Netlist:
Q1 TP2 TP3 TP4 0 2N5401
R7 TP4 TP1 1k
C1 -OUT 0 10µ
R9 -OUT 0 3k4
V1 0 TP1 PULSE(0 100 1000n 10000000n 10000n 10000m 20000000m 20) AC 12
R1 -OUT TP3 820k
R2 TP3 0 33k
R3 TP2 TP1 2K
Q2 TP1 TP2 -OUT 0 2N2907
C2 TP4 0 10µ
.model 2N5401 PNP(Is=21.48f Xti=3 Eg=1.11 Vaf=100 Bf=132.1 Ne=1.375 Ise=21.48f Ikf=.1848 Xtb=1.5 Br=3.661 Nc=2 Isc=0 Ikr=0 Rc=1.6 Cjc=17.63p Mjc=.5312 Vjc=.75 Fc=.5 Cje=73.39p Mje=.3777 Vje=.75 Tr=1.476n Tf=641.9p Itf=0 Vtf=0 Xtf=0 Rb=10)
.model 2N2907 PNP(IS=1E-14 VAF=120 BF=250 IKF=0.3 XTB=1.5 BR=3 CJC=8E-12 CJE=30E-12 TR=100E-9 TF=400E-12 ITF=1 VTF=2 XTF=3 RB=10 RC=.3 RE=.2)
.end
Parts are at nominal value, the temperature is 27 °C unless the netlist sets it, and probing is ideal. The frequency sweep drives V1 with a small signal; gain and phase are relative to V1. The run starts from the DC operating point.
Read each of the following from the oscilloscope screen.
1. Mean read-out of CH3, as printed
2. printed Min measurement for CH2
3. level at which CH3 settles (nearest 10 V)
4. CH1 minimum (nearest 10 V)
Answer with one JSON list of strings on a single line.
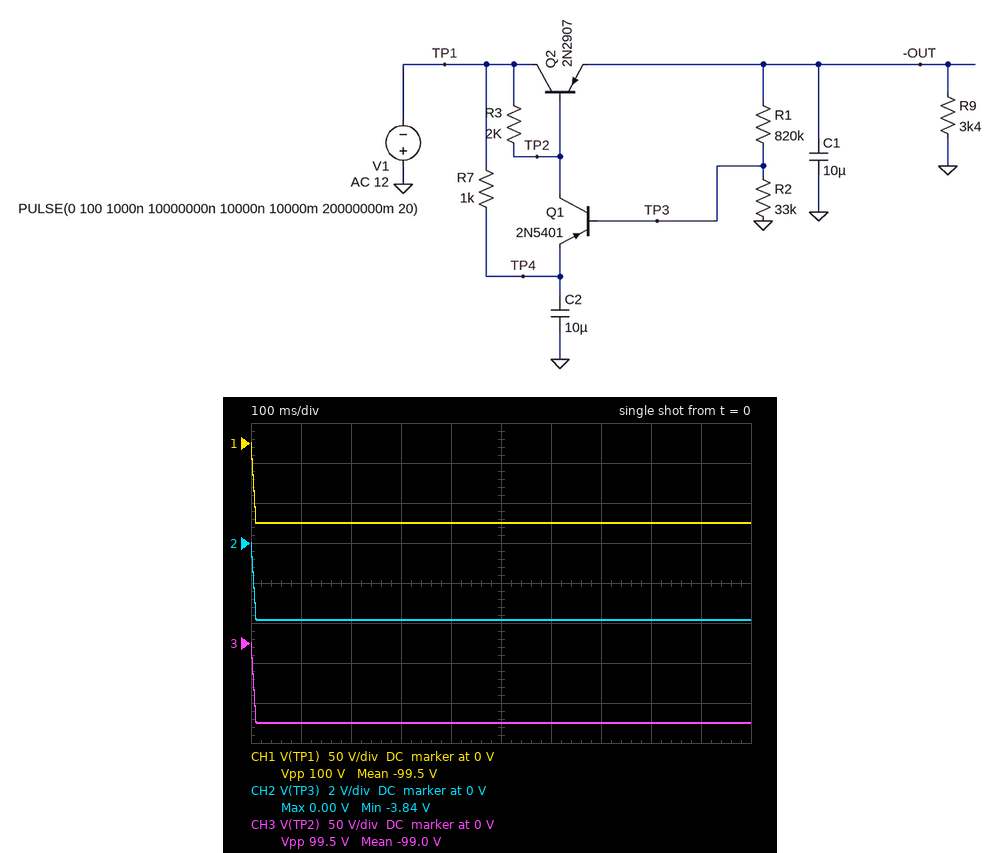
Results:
["-99.0 V", "-3.84 V", "-100 V", "-100 V"]
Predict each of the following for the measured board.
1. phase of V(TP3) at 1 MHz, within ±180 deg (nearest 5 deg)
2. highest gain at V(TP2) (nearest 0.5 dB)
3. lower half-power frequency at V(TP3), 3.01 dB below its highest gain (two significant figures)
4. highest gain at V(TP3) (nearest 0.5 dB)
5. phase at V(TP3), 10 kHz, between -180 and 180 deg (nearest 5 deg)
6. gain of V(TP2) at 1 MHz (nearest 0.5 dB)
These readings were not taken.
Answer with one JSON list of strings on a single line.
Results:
["155 deg", "0 dB", "51 kHz", "-14.5 dB", "-100 deg", "-1.5 dB"]
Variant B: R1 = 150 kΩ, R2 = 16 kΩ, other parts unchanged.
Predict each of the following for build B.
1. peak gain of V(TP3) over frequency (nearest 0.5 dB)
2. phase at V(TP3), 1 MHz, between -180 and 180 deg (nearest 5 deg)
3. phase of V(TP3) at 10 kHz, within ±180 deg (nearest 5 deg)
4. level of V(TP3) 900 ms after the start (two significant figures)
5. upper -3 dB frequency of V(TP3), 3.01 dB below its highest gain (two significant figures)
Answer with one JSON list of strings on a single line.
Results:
["-15.0 dB", "160 deg", "-95 deg", "-9.5 V", "1.8 MHz"]
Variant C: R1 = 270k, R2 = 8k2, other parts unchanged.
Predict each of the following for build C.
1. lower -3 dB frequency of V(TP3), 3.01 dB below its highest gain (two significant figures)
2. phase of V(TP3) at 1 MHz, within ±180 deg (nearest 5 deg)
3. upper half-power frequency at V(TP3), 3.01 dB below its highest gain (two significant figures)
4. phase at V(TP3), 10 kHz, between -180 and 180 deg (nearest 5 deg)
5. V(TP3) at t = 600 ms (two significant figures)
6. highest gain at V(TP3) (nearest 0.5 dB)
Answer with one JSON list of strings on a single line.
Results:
["170 kHz", "165 deg", "2.0 MHz", "-95 deg", "-2.9 V", "-15.5 dB"]
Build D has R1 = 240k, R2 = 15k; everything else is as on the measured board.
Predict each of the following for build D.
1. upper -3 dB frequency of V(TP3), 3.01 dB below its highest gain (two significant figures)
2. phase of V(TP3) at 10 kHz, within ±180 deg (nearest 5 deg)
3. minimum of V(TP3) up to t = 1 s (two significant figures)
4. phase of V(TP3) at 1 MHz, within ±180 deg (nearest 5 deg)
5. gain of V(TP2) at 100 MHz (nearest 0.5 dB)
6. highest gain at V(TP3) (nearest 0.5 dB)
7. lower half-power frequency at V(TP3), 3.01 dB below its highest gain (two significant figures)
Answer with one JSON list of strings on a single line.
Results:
["1.8 MHz", "-95 deg", "-5.8 V", "160 deg", "-16.0 dB", "-15.0 dB", "110 kHz"]
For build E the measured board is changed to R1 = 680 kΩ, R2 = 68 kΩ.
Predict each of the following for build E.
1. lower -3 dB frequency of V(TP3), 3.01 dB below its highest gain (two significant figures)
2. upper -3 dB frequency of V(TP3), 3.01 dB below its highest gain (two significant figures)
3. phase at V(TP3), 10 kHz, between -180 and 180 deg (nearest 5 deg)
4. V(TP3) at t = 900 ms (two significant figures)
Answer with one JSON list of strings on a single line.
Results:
["27 kHz", "1.6 MHz", "-110 deg", "-9.0 V"]
